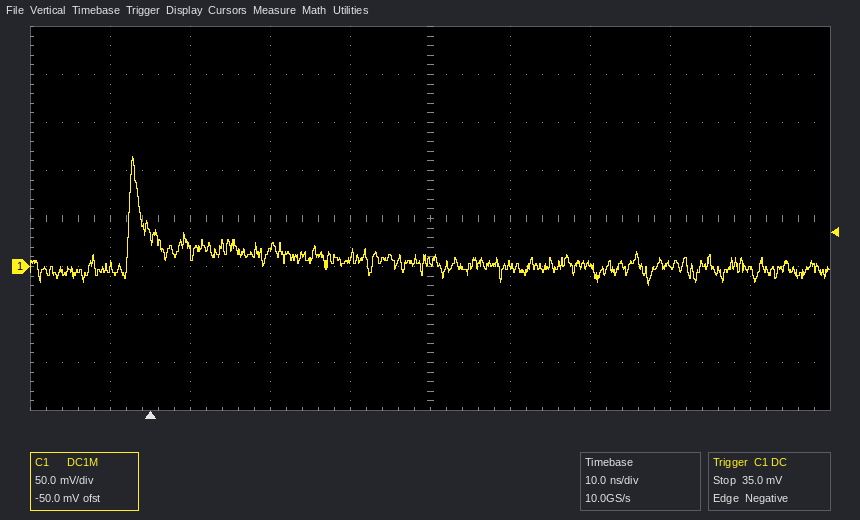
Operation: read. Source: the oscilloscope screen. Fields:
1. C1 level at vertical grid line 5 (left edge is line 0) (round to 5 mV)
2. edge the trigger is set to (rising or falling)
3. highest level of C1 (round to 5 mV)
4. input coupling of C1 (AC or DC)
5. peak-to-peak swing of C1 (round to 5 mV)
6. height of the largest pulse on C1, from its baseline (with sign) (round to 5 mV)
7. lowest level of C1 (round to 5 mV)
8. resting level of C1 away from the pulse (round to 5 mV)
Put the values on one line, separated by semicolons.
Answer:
5 mV; falling; 115 mV; DC; 135 mV; +115 mV; -20 mV; 0 mV
